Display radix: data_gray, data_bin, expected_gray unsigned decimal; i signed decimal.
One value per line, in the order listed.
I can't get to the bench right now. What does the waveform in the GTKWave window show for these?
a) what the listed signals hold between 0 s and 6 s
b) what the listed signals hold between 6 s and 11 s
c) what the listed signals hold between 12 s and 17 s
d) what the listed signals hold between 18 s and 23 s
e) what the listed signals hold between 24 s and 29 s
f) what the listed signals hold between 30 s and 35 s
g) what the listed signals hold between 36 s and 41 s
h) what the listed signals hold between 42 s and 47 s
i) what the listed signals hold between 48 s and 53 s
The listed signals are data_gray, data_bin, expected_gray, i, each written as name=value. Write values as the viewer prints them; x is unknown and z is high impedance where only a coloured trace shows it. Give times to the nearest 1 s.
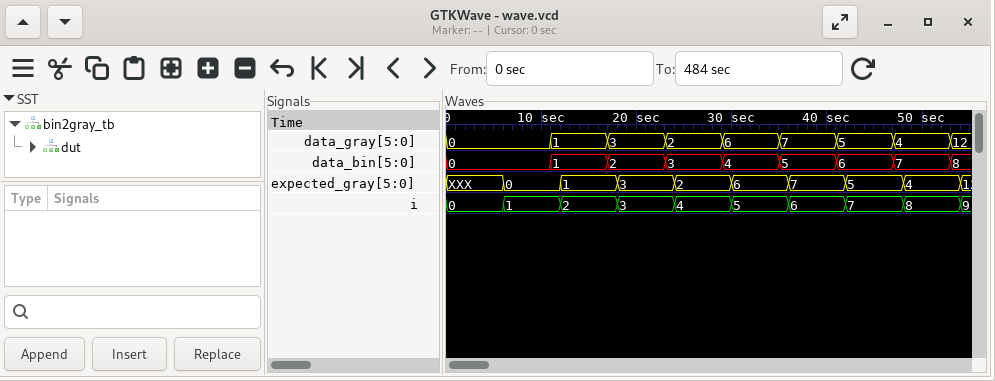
data_gray=0, data_bin=0, expected_gray=XXX, i=0
data_gray=0, data_bin=0, expected_gray=0, i=1
data_gray=1, data_bin=1, expected_gray=1, i=2
data_gray=3, data_bin=2, expected_gray=3, i=3
data_gray=2, data_bin=3, expected_gray=2, i=4
data_gray=6, data_bin=4, expected_gray=6, i=5
data_gray=7, data_bin=5, expected_gray=7, i=6
data_gray=5, data_bin=6, expected_gray=5, i=7
data_gray=4, data_bin=7, expected_gray=4, i=8
